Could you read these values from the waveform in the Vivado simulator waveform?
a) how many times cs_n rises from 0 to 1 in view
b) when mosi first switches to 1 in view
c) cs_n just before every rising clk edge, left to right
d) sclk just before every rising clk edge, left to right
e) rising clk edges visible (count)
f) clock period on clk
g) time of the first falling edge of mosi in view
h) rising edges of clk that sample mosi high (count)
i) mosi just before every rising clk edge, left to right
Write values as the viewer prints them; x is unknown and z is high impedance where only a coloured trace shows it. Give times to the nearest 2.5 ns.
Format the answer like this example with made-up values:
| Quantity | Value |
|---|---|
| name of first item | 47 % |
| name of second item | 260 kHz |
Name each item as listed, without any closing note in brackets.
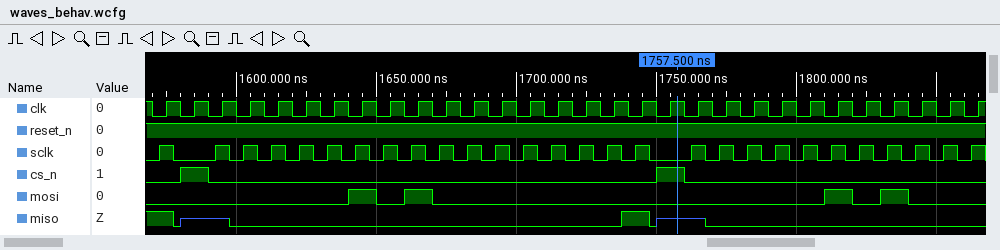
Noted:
| Quantity | Value |
|---|---|
| how many times cs_n rises from 0 to 1 in view | 2 |
| when mosi first switches to 1 in view | 1640 ns |
| cs_n just before every rising clk edge, left to right | 0 1 0 0 0 0 0 0 0 0 0 0 0 0 0 0 0 0 1 0 0 0 0 0 0 0 0 0 0 0 |
| sclk just before every rising clk edge, left to right | 1 0 1 1 1 1 1 1 1 1 1 1 1 1 1 1 1 1 0 1 1 1 1 1 1 1 1 1 1 1 |
| rising clk edges visible | 30 |
| clock period on clk | 10 ns |
| time of the first falling edge of mosi in view | 1650 ns |
| rising edges of clk that sample mosi high | 4 |
| mosi just before every rising clk edge, left to right | 0 0 0 0 0 0 0 1 0 1 0 0 0 0 0 0 0 0 0 0 0 0 0 0 1 0 1 0 0 0 |
